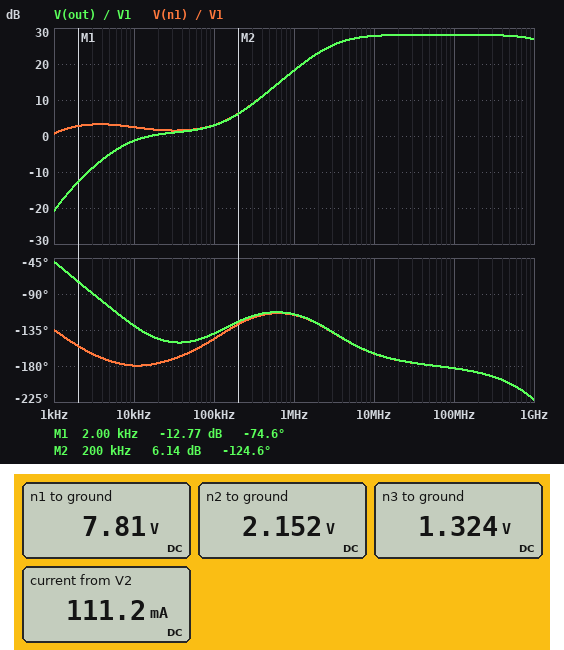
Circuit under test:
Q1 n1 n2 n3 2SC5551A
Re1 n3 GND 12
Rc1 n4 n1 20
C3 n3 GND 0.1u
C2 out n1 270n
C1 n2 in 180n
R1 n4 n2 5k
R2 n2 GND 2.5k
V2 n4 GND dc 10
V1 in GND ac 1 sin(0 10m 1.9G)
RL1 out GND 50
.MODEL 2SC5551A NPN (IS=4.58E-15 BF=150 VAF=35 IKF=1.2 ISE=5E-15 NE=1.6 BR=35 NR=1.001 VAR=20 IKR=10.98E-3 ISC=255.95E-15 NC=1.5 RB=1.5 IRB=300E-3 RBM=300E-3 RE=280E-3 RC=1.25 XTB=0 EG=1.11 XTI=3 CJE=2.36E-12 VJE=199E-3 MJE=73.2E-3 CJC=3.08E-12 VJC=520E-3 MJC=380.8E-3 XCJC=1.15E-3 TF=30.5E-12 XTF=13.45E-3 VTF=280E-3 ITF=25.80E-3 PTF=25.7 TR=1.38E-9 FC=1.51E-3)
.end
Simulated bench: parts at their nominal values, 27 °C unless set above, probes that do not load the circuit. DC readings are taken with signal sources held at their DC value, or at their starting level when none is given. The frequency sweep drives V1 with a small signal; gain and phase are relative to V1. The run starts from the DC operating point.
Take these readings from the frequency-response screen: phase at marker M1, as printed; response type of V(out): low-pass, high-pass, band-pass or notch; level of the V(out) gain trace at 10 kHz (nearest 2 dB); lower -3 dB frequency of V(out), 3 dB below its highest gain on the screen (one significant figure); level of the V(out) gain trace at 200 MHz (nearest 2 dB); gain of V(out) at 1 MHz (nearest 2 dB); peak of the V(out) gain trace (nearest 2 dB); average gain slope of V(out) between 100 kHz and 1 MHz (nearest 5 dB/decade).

-74.6 deg
high-pass
-2 dB
3 MHz
28 dB
18 dB
28 dB
15 dB/decade
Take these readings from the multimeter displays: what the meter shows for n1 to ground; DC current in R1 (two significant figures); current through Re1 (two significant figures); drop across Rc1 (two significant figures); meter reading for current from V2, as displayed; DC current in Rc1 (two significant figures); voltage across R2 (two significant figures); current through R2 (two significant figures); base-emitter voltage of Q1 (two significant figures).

7.81 V
1.6 mA
110 mA
2.2 V
111.2 mA
110 mA
2.2 V
860 µA
830 mV
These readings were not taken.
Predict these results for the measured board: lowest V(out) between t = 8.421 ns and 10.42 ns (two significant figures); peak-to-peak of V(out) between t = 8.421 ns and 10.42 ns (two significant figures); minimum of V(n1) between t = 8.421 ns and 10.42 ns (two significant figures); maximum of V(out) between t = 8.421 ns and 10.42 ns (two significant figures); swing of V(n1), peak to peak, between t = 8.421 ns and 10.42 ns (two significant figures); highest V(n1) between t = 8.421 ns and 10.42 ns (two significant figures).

-170 mV
340 mV
7.6 V
170 mV
340 mV
8.0 V
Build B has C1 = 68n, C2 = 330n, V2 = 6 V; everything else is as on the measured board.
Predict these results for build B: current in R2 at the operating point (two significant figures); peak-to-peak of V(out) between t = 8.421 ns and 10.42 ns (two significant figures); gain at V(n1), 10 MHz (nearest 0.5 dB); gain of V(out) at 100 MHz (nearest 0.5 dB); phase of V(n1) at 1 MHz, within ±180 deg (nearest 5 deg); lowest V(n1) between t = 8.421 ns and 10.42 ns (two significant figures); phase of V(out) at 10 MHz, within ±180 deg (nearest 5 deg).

570 µA
270 mV
24.5 dB
25.0 dB
-125 deg
4.8 V
-170 deg
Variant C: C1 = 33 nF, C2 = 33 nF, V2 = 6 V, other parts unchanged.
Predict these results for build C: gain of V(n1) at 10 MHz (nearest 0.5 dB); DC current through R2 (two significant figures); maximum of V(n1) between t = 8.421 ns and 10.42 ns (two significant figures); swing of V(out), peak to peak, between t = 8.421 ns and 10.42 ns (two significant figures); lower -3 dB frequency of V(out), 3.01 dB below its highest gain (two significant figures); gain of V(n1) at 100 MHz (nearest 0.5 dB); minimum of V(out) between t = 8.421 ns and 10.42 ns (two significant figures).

24.5 dB
570 µA
5.1 V
270 mV
2.1 MHz
25.0 dB
-140 mV
